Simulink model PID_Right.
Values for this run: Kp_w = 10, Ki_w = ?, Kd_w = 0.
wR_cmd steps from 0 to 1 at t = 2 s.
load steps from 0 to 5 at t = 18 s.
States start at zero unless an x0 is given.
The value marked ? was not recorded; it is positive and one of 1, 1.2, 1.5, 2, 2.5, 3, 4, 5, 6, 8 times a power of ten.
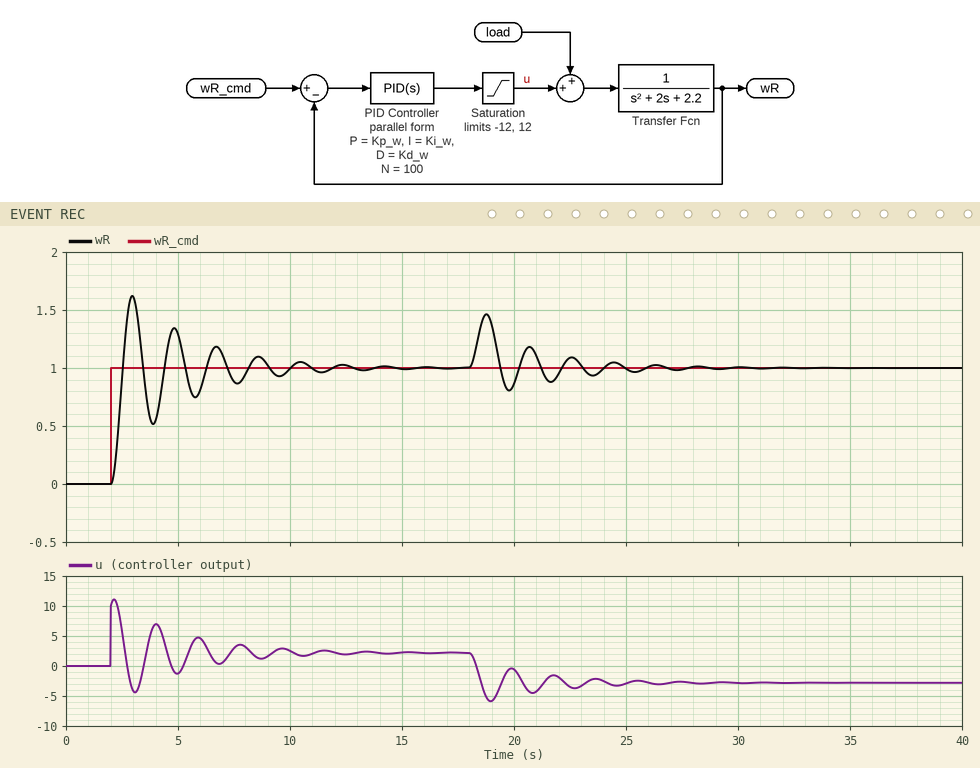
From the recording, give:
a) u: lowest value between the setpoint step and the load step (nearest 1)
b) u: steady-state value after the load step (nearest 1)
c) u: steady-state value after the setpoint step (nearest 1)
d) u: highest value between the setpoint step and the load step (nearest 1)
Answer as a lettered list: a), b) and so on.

a) -4
b) -3
c) 2
d) 11
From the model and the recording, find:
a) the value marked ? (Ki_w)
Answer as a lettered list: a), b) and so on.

a) 15
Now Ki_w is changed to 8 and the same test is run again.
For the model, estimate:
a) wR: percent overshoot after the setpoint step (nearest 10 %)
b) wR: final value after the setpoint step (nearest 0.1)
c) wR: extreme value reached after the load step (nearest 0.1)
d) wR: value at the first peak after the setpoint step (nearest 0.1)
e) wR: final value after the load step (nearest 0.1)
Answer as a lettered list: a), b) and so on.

a) 40 %
b) 1.0
c) 1.5
d) 1.4
e) 1.0
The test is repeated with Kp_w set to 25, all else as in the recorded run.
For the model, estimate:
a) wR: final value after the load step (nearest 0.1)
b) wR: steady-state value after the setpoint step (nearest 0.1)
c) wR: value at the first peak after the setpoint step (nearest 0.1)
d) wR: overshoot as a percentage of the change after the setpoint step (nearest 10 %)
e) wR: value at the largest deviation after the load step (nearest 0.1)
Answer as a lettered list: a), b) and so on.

a) 1.0
b) 1.0
c) 1.5
d) 50 %
e) 1.3
